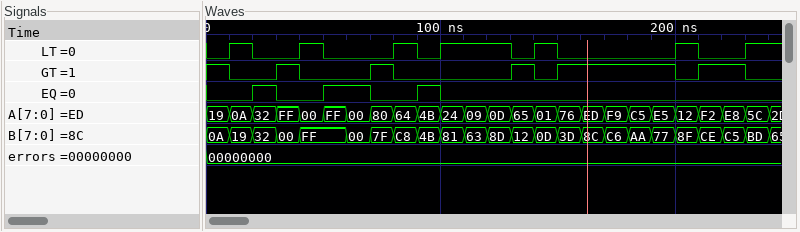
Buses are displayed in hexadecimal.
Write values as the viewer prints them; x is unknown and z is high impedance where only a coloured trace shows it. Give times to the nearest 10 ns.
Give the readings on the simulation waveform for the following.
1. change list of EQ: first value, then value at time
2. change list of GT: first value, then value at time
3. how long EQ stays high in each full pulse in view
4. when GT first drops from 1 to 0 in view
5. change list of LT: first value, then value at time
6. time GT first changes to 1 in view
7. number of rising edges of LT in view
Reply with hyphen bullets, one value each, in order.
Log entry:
- 0, 1 at 20 ns, 0 at 30 ns, 1 at 50 ns, 0 at 70 ns, 1 at 90 ns, 0 at 100 ns
- 1, 0 at 10 ns, 1 at 30 ns, 0 at 40 ns, 1 at 70 ns, 0 at 80 ns, 1 at 130 ns, 0 at 140 ns, 1 at 150 ns, 0 at 200 ns, 1 at 210 ns, 0 at 230 ns
- 10 ns, 20 ns, 10 ns
- 10 ns
- 0, 1 at 10 ns, 0 at 20 ns, 1 at 40 ns, 0 at 50 ns, 1 at 80 ns, 0 at 90 ns, 1 at 100 ns, 0 at 130 ns, 1 at 140 ns, 0 at 150 ns, 1 at 200 ns, 0 at 210 ns, 1 at 230 ns
- 30 ns
- 7
